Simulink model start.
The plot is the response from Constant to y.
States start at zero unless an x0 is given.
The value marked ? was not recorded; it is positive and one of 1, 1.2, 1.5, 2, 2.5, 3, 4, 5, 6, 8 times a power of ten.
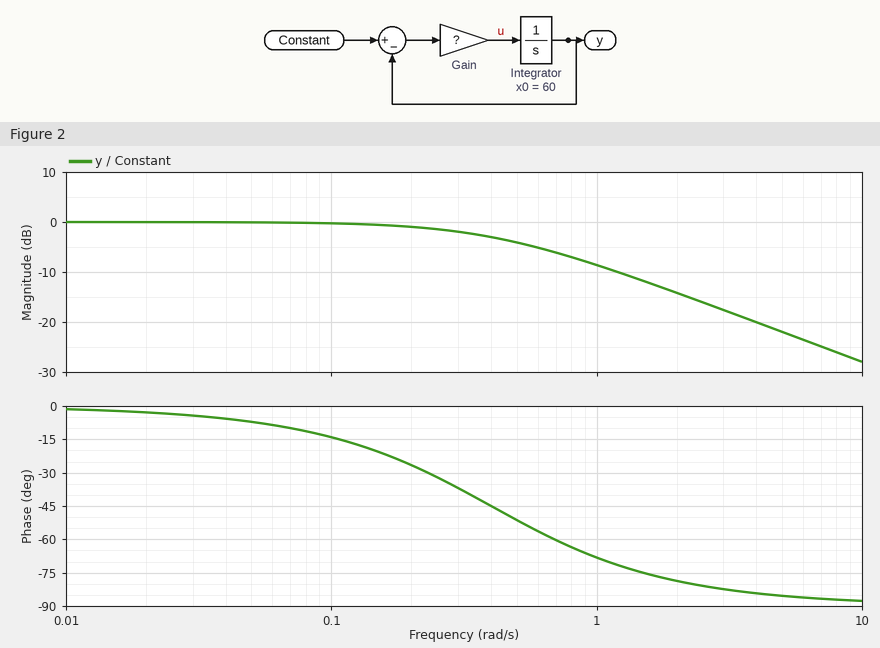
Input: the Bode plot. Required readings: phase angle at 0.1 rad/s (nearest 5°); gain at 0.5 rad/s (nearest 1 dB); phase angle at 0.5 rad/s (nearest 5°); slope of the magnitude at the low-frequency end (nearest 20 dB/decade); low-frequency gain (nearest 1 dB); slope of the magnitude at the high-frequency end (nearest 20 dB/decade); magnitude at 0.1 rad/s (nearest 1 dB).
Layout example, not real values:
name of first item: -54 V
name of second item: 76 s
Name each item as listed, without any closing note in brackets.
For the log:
phase angle at 0.1 rad/s: -15°
gain at 0.5 rad/s: -4 dB
phase angle at 0.5 rad/s: -50°
slope of the magnitude at the low-frequency end: 0 dB/decade
low-frequency gain: 0 dB
slope of the magnitude at the high-frequency end: -20 dB/decade
magnitude at 0.1 rad/s: 0 dB
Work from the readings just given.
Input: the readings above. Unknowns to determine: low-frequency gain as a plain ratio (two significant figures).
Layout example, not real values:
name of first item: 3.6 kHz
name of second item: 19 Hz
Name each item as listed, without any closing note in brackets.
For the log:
low-frequency gain as a plain ratio: 1.0
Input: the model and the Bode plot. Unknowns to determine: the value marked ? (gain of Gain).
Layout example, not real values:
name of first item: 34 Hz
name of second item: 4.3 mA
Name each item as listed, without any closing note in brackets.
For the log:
the value marked ?: 0.4
